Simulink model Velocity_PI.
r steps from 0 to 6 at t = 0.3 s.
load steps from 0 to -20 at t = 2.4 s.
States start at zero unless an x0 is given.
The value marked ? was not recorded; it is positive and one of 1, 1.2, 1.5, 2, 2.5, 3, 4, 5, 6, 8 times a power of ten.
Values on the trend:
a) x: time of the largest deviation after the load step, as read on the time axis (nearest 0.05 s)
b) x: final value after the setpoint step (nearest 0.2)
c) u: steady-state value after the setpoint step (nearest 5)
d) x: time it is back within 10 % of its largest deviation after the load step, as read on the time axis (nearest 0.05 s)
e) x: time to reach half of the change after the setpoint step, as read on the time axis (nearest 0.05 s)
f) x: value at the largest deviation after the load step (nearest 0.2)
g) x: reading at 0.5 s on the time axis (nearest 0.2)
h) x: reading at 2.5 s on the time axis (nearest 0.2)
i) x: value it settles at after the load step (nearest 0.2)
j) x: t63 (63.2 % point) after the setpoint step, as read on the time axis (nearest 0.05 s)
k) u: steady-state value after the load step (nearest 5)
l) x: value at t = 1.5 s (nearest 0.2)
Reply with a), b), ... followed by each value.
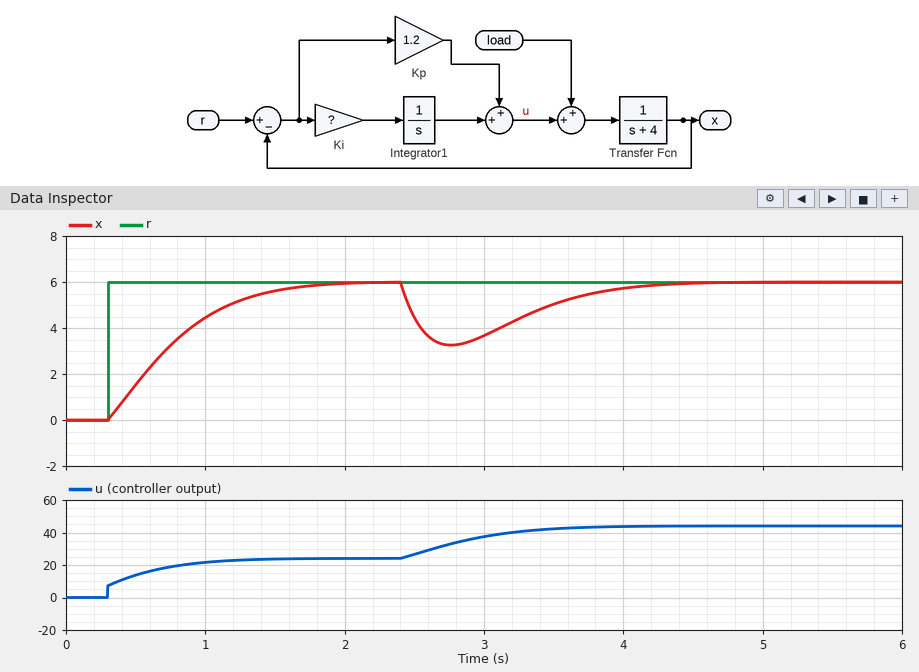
a) 2.75 s
b) 6.0
c) 25
d) 4.00 s
e) 0.70 s
f) 3.2
g) 1.6
h) 4.4
i) 6.0
j) 0.85 s
k) 45
l) 5.6
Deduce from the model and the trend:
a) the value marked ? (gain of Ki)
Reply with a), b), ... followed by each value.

a) 8
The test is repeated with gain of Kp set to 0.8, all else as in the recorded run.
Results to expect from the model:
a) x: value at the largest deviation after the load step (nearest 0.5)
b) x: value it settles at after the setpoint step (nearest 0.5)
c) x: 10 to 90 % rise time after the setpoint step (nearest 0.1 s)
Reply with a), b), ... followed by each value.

a) 3.0
b) 6.0
c) 0.9 s
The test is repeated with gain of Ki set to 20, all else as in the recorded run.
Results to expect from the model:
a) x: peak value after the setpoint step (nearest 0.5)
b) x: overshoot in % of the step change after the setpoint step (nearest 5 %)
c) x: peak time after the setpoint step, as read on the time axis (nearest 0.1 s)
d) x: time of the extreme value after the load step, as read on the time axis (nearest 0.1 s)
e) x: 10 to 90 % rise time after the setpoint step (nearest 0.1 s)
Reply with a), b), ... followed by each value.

a) 6.5
b) 10 %
c) 1.1 s
d) 2.7 s
e) 0.4 s
